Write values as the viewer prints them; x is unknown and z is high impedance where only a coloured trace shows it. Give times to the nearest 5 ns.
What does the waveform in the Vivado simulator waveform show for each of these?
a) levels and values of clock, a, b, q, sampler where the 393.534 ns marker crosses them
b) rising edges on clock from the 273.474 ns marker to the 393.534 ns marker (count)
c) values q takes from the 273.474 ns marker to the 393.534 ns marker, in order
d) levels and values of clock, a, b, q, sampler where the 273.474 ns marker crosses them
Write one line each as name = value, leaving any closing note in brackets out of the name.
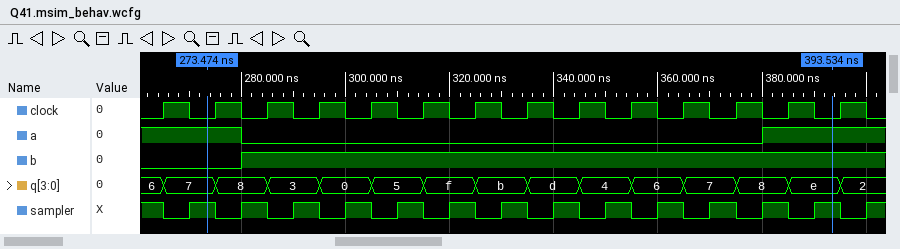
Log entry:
levels and values of clock, a, b, q, sampler where the 393.534 ns marker crosses them = clock=0, a=1, b=1, q=e, sampler=1
rising edges on clock from the 273.474 ns marker to the 393.534 ns marker = 12
values q takes from the 273.474 ns marker to the 393.534 ns marker, in order = 7, 8, 3, 0, 5, f, b, d, 4, 6, 7, 8, e
levels and values of clock, a, b, q, sampler where the 273.474 ns marker crosses them = clock=0, a=1, b=0, q=7, sampler=1
